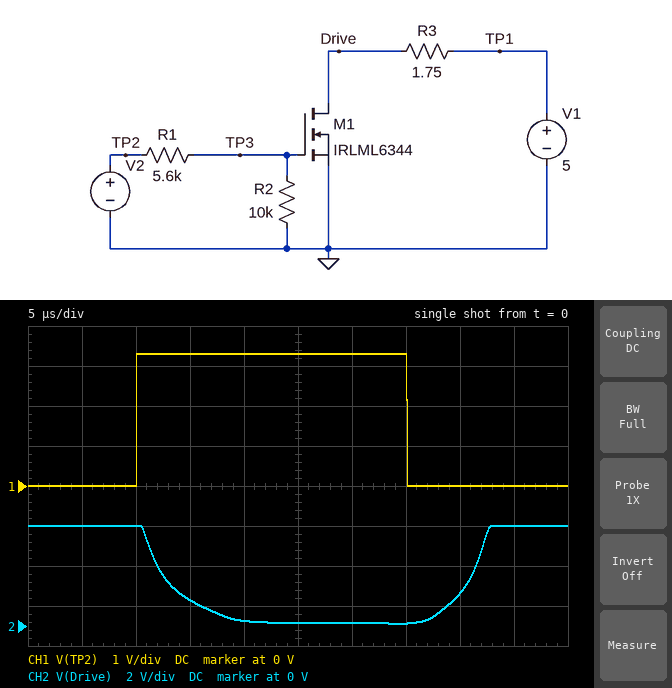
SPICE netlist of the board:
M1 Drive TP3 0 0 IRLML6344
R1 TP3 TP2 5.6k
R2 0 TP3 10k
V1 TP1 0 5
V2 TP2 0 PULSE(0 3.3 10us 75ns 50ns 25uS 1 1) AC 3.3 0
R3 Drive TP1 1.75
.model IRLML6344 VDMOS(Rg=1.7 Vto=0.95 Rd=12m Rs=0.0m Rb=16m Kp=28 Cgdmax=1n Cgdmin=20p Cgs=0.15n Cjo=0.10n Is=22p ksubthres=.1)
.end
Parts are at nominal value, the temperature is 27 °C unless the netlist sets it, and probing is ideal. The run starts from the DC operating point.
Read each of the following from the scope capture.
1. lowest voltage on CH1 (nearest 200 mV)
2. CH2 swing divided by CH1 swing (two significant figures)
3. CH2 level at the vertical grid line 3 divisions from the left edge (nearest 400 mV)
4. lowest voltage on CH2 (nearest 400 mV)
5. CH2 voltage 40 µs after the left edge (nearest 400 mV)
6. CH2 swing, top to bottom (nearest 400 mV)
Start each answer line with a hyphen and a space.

- 0 V
- 1.5
- 1.2 V
- 0 V
- 1.6 V
- 4.8 V
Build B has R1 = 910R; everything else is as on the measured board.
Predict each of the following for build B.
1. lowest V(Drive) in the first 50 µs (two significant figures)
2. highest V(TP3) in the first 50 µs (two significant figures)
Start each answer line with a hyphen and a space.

- 83 mV
- 3.0 V
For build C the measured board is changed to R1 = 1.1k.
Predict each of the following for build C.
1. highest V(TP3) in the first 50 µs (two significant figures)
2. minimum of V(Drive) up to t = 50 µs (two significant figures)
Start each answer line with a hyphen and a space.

- 3.0 V
- 84 mV
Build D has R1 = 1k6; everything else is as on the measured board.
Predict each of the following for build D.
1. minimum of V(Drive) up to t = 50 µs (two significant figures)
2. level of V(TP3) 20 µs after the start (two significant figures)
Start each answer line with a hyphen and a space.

- 87 mV
- 2.8 V
